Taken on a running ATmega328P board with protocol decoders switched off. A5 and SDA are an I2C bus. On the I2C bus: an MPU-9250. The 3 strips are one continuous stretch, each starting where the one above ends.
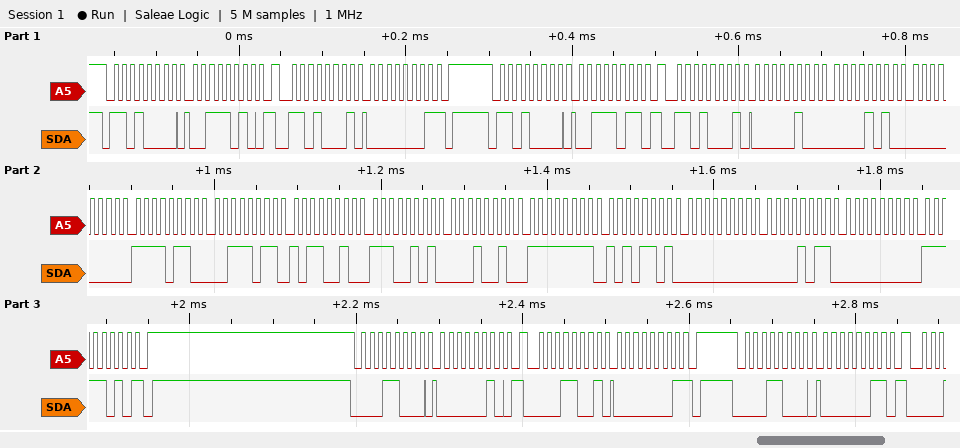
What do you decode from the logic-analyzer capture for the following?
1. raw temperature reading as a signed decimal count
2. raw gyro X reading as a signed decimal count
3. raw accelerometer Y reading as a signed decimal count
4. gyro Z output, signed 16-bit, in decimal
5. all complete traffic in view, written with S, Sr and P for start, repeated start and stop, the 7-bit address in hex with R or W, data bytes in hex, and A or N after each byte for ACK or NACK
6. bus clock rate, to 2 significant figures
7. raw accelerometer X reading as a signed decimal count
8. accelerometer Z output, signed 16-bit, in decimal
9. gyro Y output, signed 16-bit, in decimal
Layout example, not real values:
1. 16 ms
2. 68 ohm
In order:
1. -6894
2. -83
3. 246
4. 250
5. S 68W A 3A A Sr 68R A 01 N P S 68W A 3B A Sr 68R A 04 A 0A A 00 A F6 A 3B A B2 A E5 A 12 A FF A AD A 00 A 0B A 00 A FA N P S 0CW A 02 A Sr 0CR A 01 N P S 0CW A 03 A
6. 100 kHz
7. 1034
8. 15282
9. 11
